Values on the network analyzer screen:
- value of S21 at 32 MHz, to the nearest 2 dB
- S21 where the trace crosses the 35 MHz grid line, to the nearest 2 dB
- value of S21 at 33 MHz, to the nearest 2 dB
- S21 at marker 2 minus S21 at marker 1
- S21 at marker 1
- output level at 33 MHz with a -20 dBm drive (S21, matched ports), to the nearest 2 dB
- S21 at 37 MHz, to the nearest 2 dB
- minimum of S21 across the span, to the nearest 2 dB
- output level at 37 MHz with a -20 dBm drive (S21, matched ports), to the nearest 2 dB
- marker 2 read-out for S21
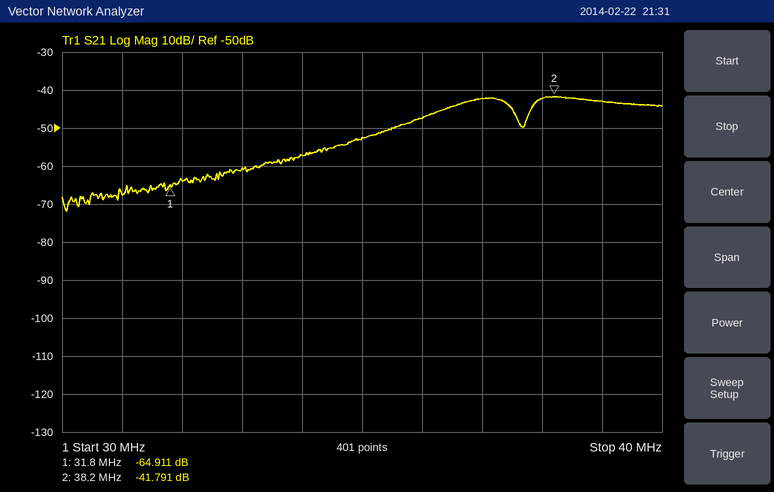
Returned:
-64 dB
-52 dB
-60 dB
23.120 dB
-64.911 dB
-80 dBm
-42 dB
-72 dB
-62 dBm
-41.791 dB
